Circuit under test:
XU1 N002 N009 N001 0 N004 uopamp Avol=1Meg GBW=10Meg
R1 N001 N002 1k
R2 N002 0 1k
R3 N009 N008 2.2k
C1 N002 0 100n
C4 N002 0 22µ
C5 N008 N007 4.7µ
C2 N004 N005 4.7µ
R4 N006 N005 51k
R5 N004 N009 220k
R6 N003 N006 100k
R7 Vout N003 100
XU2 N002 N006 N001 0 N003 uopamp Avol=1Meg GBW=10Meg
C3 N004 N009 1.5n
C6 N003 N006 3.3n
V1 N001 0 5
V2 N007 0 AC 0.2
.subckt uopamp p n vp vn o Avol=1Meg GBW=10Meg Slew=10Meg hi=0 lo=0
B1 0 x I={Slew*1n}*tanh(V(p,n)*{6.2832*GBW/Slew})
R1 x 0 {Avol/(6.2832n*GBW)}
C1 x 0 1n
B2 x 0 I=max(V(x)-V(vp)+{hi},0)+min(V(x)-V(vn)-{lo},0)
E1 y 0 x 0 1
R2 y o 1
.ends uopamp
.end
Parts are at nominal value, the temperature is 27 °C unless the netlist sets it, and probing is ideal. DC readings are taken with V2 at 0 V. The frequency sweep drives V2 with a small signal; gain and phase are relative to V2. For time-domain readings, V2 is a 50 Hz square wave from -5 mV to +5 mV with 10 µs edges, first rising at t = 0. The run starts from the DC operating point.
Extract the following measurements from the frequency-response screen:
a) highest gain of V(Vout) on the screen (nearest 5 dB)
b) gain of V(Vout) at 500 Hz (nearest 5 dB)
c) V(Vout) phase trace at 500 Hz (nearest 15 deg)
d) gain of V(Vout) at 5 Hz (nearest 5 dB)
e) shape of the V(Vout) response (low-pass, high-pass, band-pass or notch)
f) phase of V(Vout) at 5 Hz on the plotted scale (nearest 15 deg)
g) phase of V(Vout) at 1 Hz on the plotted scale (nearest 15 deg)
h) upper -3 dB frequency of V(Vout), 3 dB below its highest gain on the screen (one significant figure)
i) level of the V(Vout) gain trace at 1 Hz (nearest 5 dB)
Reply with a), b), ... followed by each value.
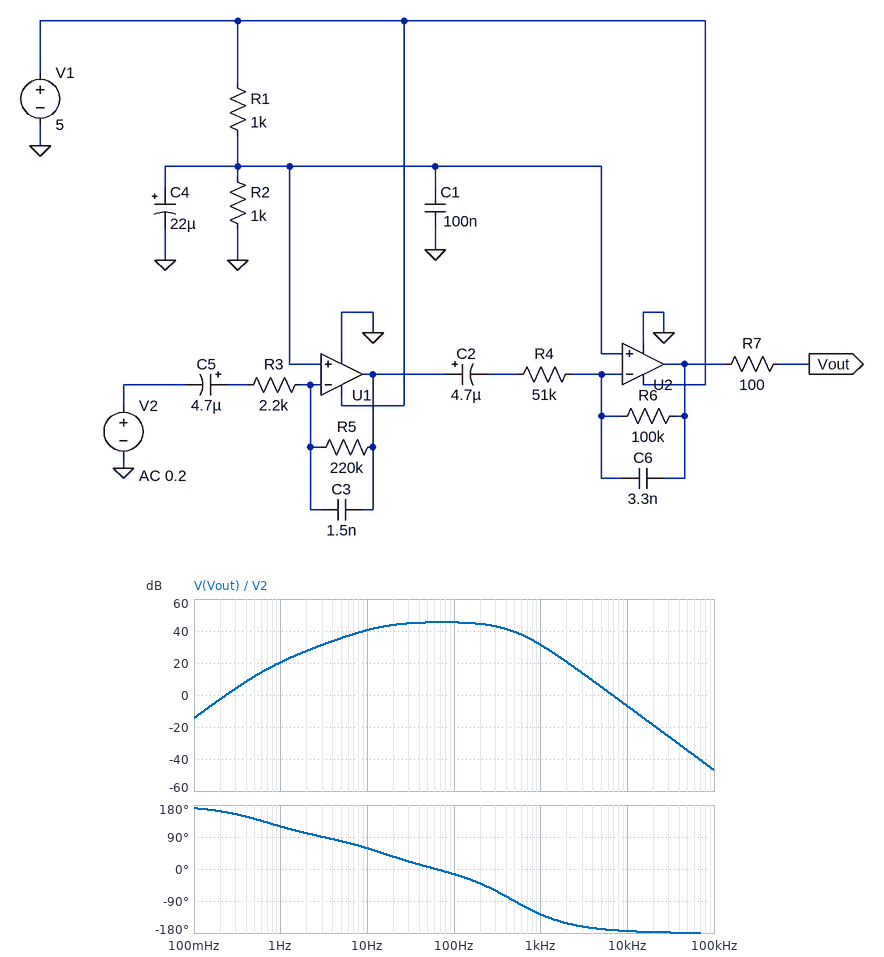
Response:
a) 45 dB
b) 40 dB
c) -90 deg
d) 35 dB
e) band-pass
f) 75 deg
g) 120 deg
h) 300 Hz
i) 20 dB
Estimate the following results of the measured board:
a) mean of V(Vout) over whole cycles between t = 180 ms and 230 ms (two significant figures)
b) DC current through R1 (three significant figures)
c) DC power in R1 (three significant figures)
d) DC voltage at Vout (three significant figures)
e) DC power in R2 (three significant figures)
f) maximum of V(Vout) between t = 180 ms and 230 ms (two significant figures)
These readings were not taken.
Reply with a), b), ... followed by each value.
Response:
a) 2.5 V
b) 2.50 mA
c) 6.25 mW
d) 2.50 V
e) 6.25 mW
f) 3.7 V
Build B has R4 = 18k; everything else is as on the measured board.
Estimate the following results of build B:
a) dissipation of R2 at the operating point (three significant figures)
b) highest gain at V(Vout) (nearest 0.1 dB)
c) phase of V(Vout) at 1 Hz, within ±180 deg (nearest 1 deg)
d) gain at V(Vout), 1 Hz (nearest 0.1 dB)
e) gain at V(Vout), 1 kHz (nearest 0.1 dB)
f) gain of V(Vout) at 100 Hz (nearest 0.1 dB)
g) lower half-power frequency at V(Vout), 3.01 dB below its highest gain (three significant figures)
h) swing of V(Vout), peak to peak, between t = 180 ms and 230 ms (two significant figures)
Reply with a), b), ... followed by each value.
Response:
a) 6.25 mW
b) 54.5 dB
c) 148 deg
d) 24.6 dB
e) 40.4 dB
f) 54.4 dB
g) 14.4 Hz
h) 5.0 V
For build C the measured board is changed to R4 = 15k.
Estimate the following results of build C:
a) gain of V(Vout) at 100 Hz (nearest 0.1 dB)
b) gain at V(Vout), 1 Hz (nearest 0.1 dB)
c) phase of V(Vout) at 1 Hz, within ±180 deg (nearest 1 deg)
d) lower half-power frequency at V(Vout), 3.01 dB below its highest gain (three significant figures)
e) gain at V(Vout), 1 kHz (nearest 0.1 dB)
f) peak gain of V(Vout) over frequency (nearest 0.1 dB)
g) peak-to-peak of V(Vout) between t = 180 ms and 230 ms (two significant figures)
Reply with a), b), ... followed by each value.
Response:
a) 56.0 dB
b) 24.9 dB
c) 152 deg
d) 14.5 Hz
e) 42.0 dB
f) 56.1 dB
g) 5.0 V
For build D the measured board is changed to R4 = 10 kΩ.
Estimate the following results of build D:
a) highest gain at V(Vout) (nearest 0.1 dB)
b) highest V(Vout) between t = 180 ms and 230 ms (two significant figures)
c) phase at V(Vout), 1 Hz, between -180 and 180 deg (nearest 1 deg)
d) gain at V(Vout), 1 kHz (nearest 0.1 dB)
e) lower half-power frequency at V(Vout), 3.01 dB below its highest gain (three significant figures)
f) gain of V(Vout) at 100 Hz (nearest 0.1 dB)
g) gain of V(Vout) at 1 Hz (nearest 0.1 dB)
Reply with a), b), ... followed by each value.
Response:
a) 59.6 dB
b) 5.0 V
c) 160 deg
d) 45.5 dB
e) 14.8 Hz
f) 59.5 dB
g) 25.3 dB
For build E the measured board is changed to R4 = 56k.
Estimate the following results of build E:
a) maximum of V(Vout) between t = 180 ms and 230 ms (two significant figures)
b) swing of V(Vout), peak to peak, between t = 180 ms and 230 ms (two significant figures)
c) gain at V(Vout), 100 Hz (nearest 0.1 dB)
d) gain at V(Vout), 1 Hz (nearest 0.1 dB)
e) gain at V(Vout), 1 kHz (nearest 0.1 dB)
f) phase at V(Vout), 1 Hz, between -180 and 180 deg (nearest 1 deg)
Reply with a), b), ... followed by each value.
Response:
a) 3.6 V
b) 2.2 V
c) 44.6 dB
d) 19.9 dB
e) 30.5 dB
f) 117 deg
